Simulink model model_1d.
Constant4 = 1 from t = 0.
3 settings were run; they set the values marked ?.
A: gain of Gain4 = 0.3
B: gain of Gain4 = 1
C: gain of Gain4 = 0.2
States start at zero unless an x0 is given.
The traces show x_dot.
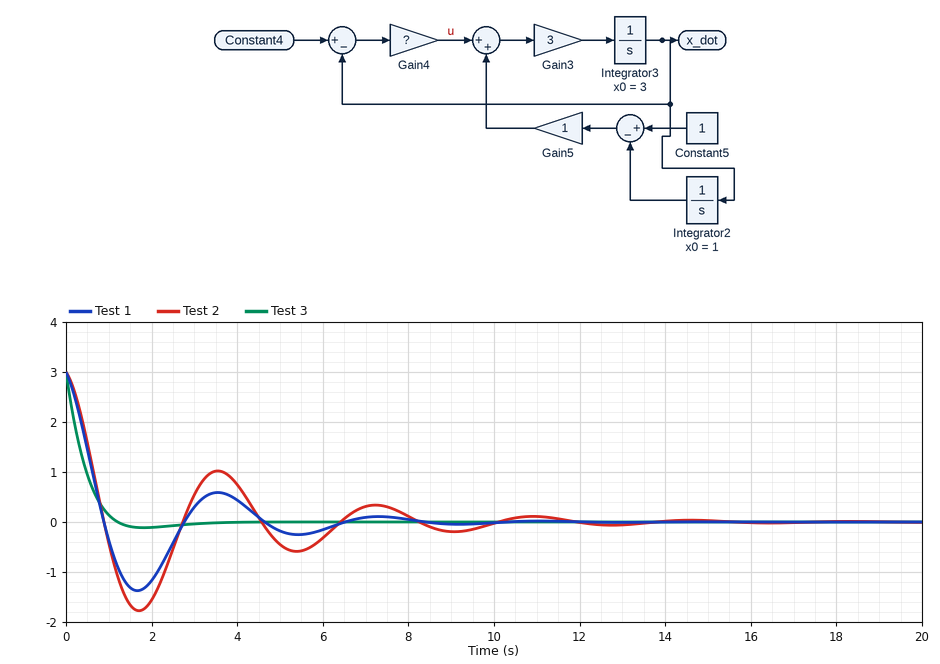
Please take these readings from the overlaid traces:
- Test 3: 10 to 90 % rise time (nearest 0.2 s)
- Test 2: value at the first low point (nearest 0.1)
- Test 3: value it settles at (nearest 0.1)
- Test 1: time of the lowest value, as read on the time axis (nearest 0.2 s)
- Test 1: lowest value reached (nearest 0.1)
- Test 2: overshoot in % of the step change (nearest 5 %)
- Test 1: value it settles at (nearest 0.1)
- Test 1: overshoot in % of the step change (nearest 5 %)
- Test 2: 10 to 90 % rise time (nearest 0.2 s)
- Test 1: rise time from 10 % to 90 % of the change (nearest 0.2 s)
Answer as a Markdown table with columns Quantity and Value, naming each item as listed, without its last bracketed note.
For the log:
| Quantity | Value |
|---|---|
| Test 3: 10 to 90 % rise time | 0.8 s |
| Test 2: value at the first low point | -1.8 |
| Test 3: value it settles at | 0.0 |
| Test 1: time of the lowest value, as read on the time axis | 1.6 s |
| Test 1: lowest value reached | -1.4 |
| Test 2: overshoot in % of the step change | 60 % |
| Test 1: value it settles at | 0.0 |
| Test 1: overshoot in % of the step change | 45 % |
| Test 2: 10 to 90 % rise time | 0.6 s |
| Test 1: rise time from 10 % to 90 % of the change | 0.6 s |
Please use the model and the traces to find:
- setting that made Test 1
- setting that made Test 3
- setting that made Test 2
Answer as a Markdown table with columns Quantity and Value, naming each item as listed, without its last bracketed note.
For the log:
| Quantity | Value |
|---|---|
| setting that made Test 1 | A |
| setting that made Test 3 | B |
| setting that made Test 2 | C |
